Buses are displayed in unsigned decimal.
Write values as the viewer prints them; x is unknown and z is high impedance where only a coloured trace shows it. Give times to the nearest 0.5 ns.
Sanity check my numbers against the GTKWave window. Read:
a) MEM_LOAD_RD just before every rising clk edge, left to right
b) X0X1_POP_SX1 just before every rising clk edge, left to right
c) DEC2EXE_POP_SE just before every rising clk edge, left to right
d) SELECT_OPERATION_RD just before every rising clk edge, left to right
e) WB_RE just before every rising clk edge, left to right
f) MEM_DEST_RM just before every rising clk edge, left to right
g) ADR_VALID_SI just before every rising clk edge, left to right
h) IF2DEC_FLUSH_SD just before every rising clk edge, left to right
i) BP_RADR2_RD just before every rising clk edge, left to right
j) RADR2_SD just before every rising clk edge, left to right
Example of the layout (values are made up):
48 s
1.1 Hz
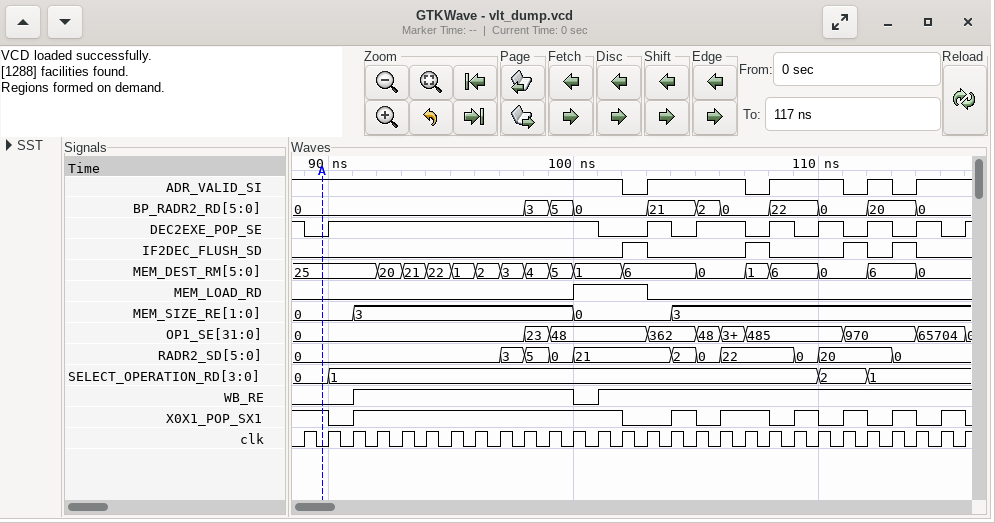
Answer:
0 0 0 0 0 0 0 0 0 0 0 0 1 1 1 0 0 0 0 0 0 0 0 0 0 0 0 0
1 1 0 1 1 1 1 1 1 1 1 1 1 1 0 0 1 0 1 1 0 1 0 1 0 1 0 1
1 0 1 1 1 1 1 1 1 1 1 1 1 0 0 1 0 1 1 0 1 0 1 0 1 0 1 0
0, 0, 1, 1, 1, 1, 1, 1, 1, 1, 1, 1, 1, 1, 1, 1, 1, 1, 1, 1, 1, 1, 2, 2, 1, 1, 1, 1
0 0 0 1 1 1 1 1 1 1 1 1 0 1 1 1 1 1 1 1 1 1 1 1 1 1 1 1
25, 25, 25, 25, 20, 21, 22, 1, 2, 3, 4, 5, 1, 1, 6, 6, 6, 0, 0, 1, 6, 6, 0, 0, 6, 6, 0, 0
1 1 1 1 1 1 1 1 1 1 1 1 1 1 0 1 1 1 1 0 1 1 1 0 1 0 1 1
0 0 0 0 0 0 0 0 0 0 0 0 0 0 1 0 0 0 0 1 0 0 0 1 0 1 0 0
0, 0, 0, 0, 0, 0, 0, 0, 0, 0, 3, 5, 0, 0, 0, 21, 21, 2, 0, 0, 22, 22, 0, 0, 20, 20, 0, 0
0, 0, 0, 0, 0, 0, 0, 0, 0, 3, 5, 0, 21, 21, 21, 21, 2, 0, 22, 22, 22, 0, 20, 20, 20, 0, 0, 0
